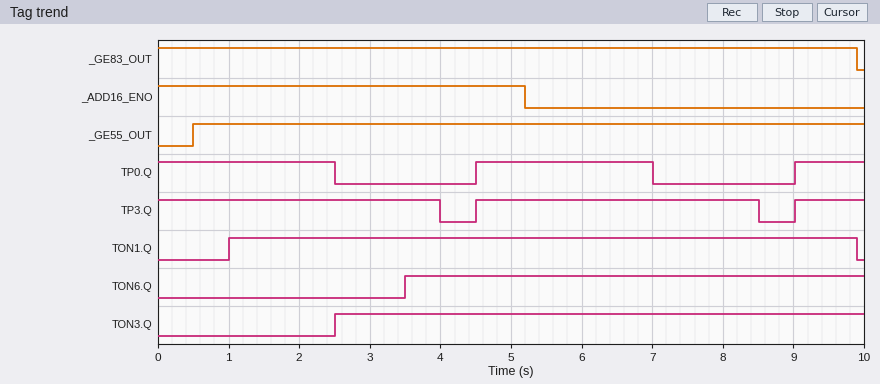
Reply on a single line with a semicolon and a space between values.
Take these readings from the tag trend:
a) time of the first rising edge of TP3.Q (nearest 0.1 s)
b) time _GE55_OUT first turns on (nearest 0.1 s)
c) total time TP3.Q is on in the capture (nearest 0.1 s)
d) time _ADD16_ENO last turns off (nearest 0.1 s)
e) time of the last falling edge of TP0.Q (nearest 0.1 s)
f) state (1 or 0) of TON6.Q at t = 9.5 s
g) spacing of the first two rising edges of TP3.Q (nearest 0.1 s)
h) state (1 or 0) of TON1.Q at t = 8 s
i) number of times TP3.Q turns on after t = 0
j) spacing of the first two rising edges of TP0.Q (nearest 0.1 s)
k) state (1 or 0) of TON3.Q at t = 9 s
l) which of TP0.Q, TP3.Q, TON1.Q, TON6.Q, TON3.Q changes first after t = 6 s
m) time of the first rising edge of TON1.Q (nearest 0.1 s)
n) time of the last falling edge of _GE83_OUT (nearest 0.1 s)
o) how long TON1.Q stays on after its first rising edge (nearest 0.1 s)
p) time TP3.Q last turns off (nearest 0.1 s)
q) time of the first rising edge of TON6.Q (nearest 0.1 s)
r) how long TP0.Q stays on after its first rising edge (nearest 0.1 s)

4.5 s; 0.5 s; 9.0 s; 5.2 s; 7.0 s; 1; 4.5 s; 1; 2; 4.5 s; 1; TP0.Q; 1.0 s; 9.9 s; 8.9 s; 8.5 s; 3.5 s; 2.5 s
